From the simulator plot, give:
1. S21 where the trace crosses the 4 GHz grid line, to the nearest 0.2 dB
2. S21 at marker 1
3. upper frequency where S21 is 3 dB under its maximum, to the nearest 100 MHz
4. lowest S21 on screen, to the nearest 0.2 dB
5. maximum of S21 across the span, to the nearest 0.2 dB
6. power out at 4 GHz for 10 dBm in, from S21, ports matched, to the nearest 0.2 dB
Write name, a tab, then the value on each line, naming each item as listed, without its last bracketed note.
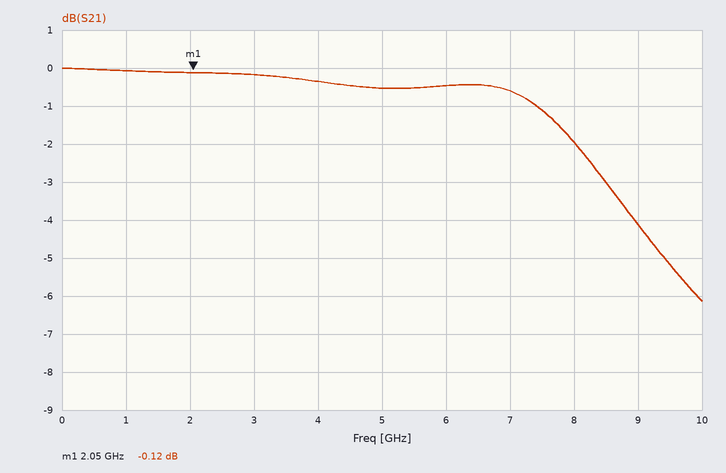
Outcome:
S21 where the trace crosses the 4 GHz grid line, to the nearest 0.2 dB	-0.4 dB
S21 at marker 1	-0.12 dB
upper frequency where S21 is 3 dB under its maximum, to the nearest 100 MHz	8.5 GHz
lowest S21 on screen, to the nearest 0.2 dB	-6.2 dB
maximum of S21 across the span, to the nearest 0.2 dB	0.0 dB
power out at 4 GHz for 10 dBm in, from S21, ports matched, to the nearest 0.2 dB	9.6 dBm
